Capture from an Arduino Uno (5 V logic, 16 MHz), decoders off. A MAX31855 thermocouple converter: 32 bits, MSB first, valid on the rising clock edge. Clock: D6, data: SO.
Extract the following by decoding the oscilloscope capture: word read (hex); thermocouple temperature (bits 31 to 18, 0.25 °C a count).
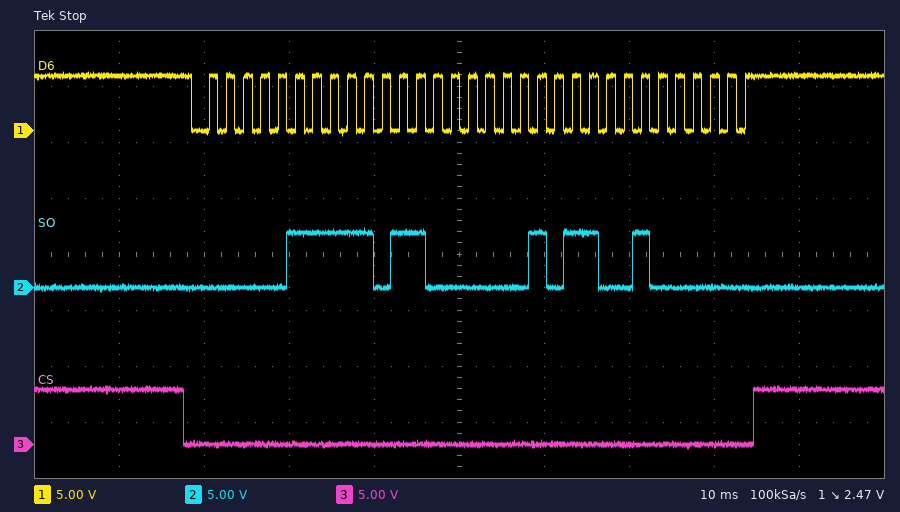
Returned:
0x07D81640
125.50 °C
